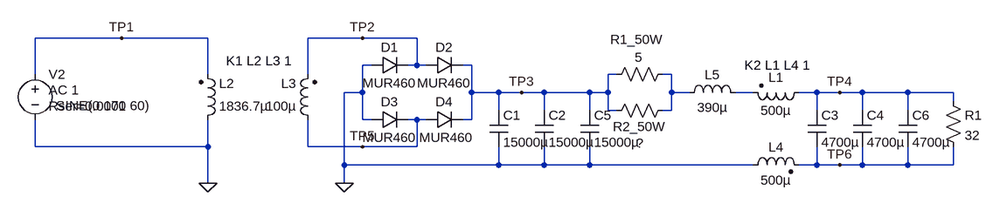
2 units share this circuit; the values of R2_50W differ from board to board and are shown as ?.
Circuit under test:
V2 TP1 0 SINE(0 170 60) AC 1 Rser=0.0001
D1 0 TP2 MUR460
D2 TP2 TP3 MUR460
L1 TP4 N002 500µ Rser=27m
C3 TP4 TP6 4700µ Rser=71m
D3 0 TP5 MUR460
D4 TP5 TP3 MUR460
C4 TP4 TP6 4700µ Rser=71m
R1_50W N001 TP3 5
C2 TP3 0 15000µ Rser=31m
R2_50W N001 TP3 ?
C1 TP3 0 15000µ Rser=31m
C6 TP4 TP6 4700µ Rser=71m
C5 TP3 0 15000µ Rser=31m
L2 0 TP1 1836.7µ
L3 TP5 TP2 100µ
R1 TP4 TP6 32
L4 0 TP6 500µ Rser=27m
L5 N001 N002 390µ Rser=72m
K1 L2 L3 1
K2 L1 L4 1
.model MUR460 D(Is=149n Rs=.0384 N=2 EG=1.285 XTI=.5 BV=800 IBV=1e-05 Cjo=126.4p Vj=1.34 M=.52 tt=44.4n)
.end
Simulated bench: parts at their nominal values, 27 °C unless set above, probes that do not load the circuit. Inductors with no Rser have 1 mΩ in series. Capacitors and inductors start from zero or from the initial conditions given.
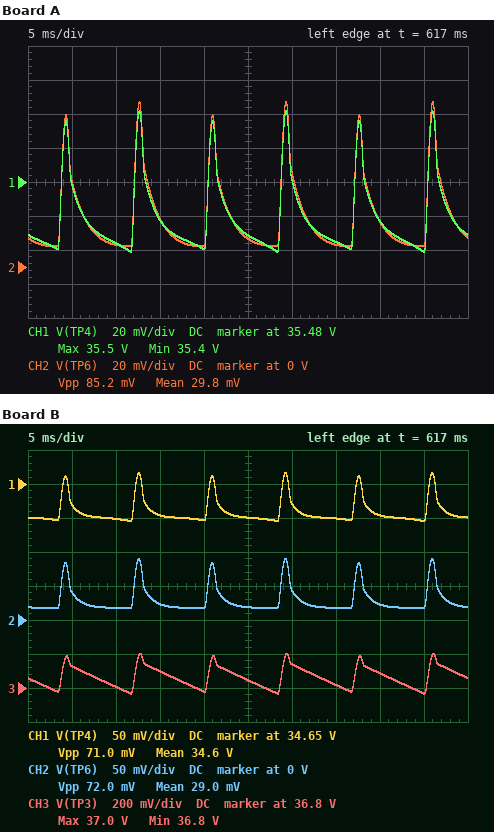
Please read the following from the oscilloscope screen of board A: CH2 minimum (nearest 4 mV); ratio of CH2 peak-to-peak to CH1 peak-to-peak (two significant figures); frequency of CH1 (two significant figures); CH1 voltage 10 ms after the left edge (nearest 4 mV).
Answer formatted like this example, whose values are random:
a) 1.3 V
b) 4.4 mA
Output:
a) 12 mV
b) 1.0
c) 120 Hz
d) 35.444 V
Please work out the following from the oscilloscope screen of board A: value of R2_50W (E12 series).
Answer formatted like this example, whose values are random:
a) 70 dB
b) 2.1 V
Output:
a) 1.5 Ω
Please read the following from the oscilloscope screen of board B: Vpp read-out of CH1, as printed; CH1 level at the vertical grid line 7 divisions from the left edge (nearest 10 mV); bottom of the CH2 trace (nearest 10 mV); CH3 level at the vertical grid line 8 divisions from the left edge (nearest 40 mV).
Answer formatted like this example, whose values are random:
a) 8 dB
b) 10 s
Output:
a) 71.0 mV
b) 34.60 V
c) 20 mV
d) 36.88 V
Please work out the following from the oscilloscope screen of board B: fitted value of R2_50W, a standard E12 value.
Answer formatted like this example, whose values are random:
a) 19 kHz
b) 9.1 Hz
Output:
a) 3.3 Ω
